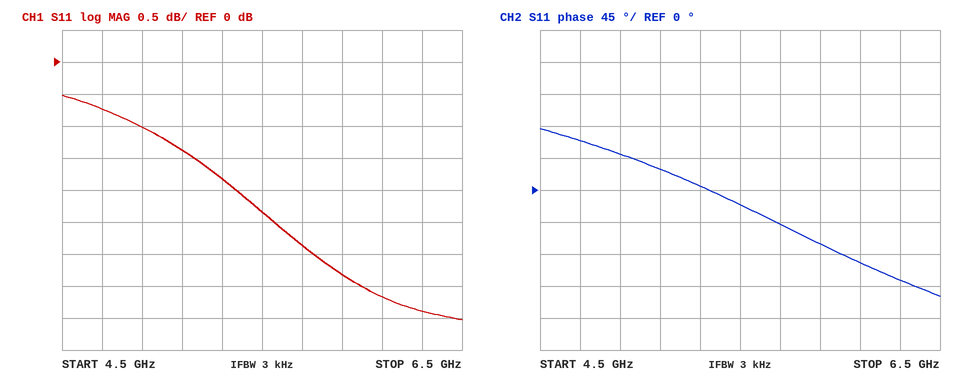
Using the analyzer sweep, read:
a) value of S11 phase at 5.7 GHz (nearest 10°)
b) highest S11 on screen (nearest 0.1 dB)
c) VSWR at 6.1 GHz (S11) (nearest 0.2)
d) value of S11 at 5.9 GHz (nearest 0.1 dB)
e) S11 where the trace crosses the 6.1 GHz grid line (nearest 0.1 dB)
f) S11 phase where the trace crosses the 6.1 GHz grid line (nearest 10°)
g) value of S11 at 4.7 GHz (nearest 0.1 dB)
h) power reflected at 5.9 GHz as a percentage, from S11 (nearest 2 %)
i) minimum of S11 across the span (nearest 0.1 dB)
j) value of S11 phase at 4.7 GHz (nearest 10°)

-50°
-0.5 dB
4.8
-3.3 dB
-3.7 dB
-100°
-0.7 dB
46 %
-4.0 dB
70°
